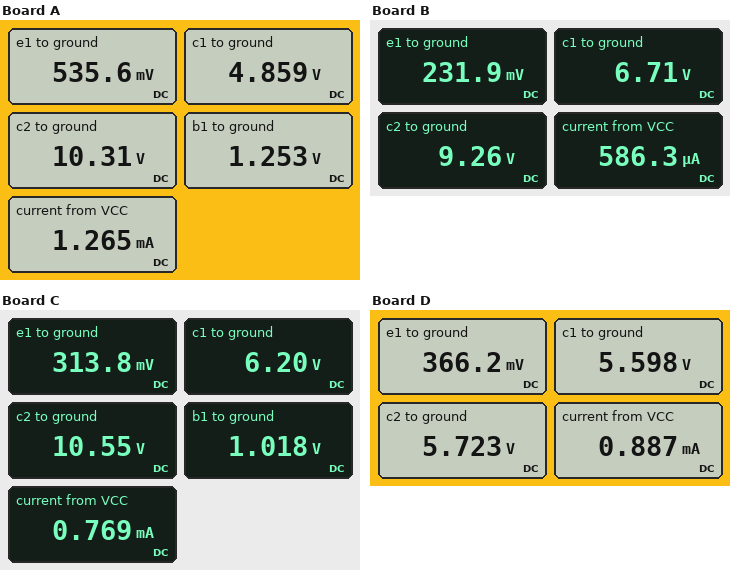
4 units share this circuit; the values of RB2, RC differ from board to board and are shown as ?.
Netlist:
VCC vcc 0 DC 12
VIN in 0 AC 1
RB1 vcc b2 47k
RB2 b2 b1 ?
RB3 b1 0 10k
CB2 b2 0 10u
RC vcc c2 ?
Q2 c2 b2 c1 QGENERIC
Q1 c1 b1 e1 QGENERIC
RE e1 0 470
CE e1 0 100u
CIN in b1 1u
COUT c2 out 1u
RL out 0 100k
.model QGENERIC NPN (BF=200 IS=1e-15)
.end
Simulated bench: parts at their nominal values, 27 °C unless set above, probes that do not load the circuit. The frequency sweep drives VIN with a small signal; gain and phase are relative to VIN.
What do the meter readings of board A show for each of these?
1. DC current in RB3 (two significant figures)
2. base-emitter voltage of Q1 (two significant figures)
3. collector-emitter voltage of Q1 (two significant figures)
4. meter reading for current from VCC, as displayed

130 µA
720 mV
4.3 V
1.265 mA
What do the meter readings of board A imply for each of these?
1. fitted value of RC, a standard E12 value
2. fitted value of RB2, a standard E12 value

1.5 kΩ
33 kΩ
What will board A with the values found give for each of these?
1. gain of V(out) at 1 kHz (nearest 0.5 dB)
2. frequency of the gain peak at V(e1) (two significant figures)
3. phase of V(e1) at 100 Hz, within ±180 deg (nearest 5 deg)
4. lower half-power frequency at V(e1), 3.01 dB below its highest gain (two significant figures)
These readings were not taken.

36.0 dB
41 Hz
-35 deg
12 Hz
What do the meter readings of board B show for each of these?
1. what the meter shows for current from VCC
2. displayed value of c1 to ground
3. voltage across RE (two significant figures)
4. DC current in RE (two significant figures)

586.3 µA
6.71 V
230 mV
490 µA
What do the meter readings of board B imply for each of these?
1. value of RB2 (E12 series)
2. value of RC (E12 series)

68 kΩ
5.6 kΩ
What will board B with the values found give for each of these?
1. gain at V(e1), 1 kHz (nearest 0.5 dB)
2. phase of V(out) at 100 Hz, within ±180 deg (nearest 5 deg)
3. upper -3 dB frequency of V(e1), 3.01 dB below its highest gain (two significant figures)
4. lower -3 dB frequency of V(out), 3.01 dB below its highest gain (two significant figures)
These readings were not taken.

-30.5 dB
-145 deg
76 Hz
57 Hz
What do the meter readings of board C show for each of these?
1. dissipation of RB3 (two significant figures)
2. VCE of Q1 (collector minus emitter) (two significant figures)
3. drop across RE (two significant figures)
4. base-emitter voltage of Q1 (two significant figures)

100 µW
5.9 V
310 mV
700 mV
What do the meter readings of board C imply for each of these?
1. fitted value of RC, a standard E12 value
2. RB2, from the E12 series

2.2 kΩ
56 kΩ
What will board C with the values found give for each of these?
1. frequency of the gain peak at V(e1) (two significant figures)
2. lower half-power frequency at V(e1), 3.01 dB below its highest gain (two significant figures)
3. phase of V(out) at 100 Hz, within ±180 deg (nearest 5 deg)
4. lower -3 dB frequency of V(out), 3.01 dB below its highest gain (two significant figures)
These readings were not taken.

30 Hz
9.7 Hz
-140 deg
73 Hz
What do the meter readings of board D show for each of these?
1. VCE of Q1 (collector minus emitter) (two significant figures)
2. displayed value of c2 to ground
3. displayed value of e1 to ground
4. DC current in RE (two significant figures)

5.2 V
5.723 V
366.2 mV
780 µA
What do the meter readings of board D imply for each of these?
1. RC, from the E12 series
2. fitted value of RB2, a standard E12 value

8.2 kΩ
47 kΩ
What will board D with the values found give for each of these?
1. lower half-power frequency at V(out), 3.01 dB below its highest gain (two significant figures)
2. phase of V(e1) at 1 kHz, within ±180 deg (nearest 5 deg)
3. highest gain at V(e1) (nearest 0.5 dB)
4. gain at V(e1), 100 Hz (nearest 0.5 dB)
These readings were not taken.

74 Hz
-85 deg
-6.0 dB
-8.0 dB
